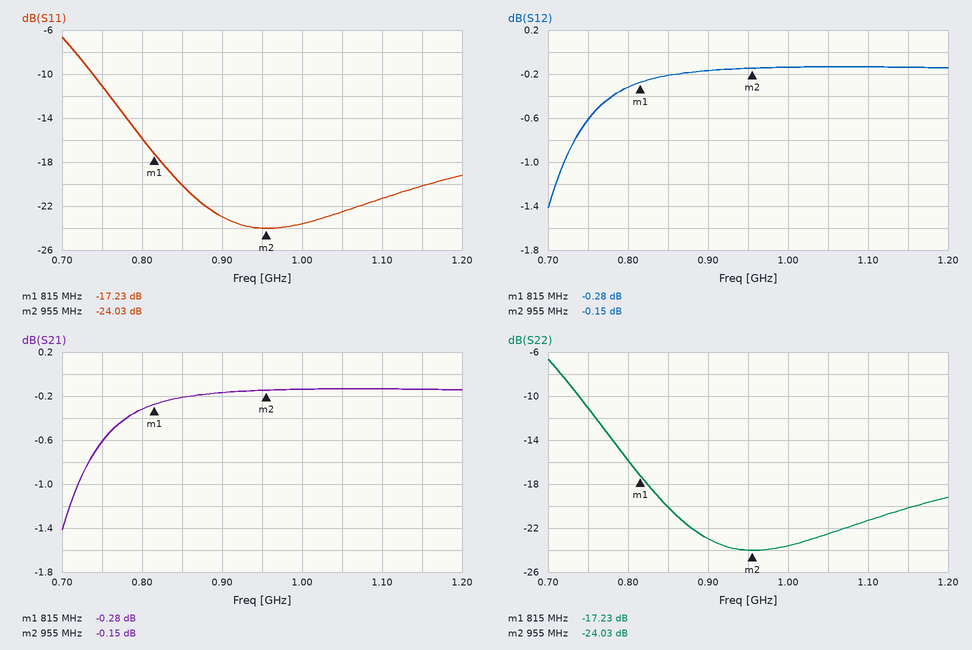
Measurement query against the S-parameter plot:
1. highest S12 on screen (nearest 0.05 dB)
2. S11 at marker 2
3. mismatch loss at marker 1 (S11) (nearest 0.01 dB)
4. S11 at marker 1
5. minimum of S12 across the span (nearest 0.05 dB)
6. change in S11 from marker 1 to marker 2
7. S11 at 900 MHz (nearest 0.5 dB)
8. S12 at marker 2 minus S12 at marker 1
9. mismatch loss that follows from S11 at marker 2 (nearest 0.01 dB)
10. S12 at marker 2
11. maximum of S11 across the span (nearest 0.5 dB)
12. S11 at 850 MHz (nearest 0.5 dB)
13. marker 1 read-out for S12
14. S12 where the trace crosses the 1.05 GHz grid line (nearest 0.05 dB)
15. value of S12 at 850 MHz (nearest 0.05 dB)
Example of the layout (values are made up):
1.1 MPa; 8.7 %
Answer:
-0.15 dB; -24.03 dB; 0.08 dB; -17.23 dB; -1.40 dB; -6.80 dB; -23.0 dB; 0.13 dB; 0.02 dB; -0.15 dB; -6.5 dB; -20.0 dB; -0.28 dB; -0.15 dB; -0.20 dB
